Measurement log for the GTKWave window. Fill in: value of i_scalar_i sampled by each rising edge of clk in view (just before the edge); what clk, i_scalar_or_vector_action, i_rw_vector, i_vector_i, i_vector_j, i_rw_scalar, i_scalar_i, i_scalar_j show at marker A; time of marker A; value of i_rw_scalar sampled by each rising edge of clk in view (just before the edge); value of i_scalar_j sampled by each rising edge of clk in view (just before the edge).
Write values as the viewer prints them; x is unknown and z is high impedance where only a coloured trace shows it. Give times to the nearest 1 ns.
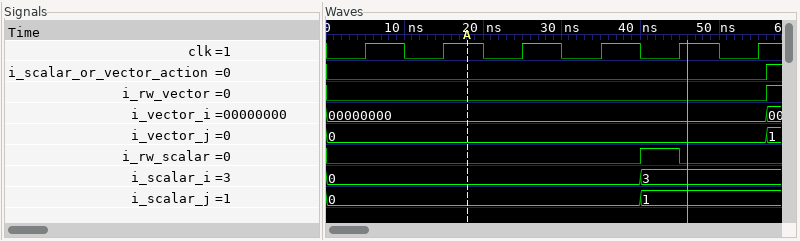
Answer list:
0, 0, 0, 0, 3, 3
clk=1, i_scalar_or_vector_action=0, i_rw_vector=0, i_vector_i=00000000, i_vector_j=0, i_rw_scalar=0, i_scalar_i=0, i_scalar_j=0
18 ns
0 0 0 0 1 0
0, 0, 0, 0, 1, 1
